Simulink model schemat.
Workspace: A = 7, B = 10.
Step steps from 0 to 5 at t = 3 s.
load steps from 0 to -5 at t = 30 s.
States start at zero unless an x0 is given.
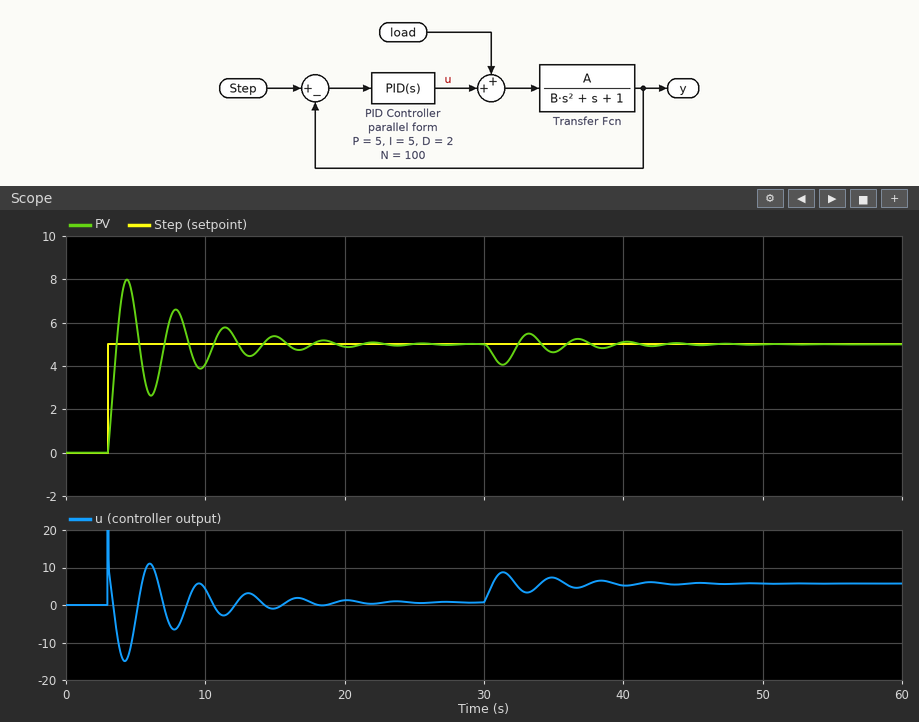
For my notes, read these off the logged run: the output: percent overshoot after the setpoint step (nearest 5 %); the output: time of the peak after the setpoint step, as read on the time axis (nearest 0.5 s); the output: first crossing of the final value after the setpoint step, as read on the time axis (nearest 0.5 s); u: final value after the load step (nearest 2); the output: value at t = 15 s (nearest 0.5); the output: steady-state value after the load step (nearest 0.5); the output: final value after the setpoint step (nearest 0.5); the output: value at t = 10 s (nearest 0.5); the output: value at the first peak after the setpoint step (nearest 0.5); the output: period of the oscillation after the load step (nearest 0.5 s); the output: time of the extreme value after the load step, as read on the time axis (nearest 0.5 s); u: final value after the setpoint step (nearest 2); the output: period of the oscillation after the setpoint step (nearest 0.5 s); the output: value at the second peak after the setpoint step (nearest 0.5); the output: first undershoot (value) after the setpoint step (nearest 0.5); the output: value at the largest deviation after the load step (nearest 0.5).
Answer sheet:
60 %
4.5 s
3.5 s
6
5.5
5.0
5.0
4.0
8.0
3.5 s
31.5 s
0
3.5 s
6.5
2.5
4.0
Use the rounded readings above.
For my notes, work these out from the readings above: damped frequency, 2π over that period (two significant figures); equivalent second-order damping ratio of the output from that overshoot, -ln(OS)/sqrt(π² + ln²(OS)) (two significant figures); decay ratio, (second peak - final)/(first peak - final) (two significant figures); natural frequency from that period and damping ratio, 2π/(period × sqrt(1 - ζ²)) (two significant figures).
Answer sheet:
1.8 rad/s
0.16
0.50
1.8 rad/s
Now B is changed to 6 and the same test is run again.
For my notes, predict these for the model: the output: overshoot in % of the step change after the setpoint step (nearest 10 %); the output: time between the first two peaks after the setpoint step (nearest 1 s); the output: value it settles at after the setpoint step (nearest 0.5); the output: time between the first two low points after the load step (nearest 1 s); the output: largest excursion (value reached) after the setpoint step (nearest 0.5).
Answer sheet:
40 %
3 s
5.0
3 s
7.0
